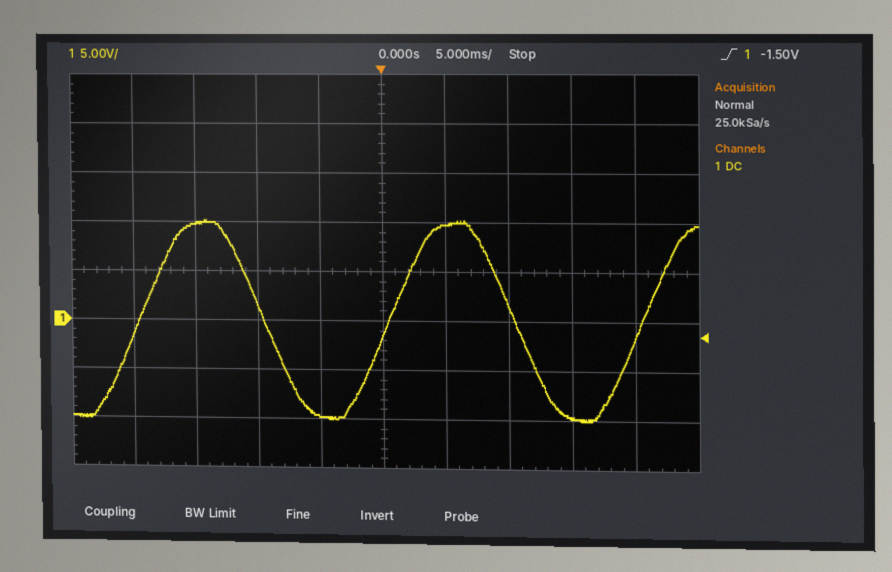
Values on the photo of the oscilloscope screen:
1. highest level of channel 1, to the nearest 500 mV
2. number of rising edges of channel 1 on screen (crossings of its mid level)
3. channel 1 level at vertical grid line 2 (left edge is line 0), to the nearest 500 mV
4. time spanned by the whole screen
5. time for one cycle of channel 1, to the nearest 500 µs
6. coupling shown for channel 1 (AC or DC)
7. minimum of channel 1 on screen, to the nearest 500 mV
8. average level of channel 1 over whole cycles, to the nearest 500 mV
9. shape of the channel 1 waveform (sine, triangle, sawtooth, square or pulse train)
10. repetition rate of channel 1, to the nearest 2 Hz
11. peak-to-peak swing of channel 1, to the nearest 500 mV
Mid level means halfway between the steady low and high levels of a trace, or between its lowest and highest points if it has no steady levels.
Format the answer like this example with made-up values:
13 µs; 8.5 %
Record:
10.0 V; 3; 10.0 V; 50 ms; 20.0 ms; DC; -10.0 V; 0.0 V; sine; 50 Hz; 20.0 V
